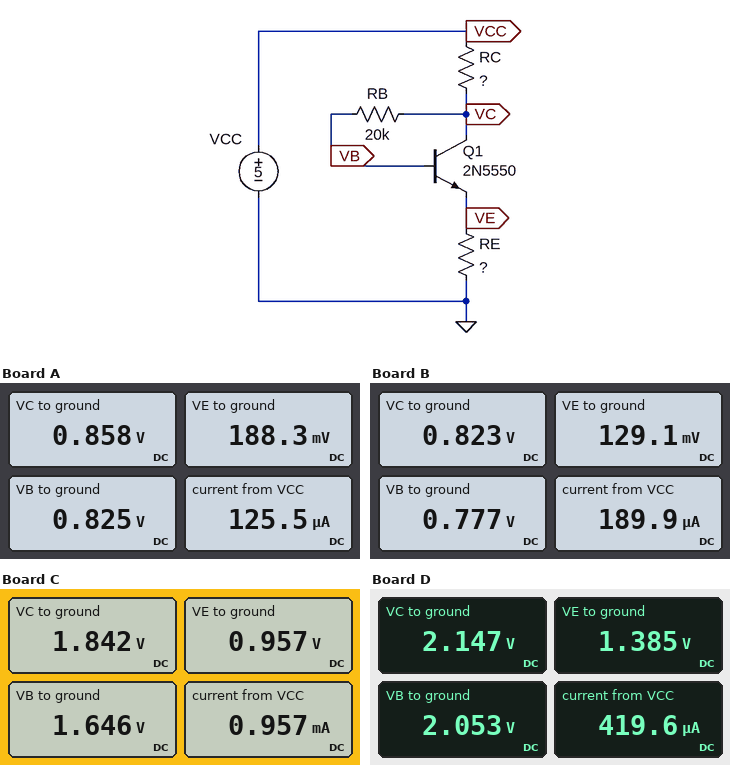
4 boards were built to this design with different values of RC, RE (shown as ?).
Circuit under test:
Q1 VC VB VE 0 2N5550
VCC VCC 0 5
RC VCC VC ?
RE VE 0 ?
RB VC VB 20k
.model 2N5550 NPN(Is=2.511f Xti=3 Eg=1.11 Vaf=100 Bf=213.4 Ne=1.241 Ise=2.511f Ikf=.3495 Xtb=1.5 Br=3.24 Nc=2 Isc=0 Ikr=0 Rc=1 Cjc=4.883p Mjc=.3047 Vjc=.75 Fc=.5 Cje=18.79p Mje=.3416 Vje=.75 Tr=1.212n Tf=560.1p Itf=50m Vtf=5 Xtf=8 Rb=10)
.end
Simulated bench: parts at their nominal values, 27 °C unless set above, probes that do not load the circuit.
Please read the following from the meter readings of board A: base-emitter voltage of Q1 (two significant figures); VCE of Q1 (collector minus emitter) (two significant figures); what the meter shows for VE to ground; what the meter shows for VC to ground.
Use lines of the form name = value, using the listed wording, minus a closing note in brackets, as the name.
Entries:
base-emitter voltage of Q1 = 640 mV
VCE of Q1 (collector minus emitter) = 670 mV
what the meter shows for VE to ground = 188.3 mV
what the meter shows for VC to ground = 0.858 V
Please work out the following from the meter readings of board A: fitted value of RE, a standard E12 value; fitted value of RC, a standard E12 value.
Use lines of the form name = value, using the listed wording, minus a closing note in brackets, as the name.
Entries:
fitted value of RE, a standard E12 value = 1.5 kΩ
fitted value of RC, a standard E12 value = 33 kΩ
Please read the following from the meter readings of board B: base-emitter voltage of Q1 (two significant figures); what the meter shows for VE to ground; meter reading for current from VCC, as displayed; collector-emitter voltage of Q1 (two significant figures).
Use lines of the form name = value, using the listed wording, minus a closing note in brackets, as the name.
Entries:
base-emitter voltage of Q1 = 650 mV
what the meter shows for VE to ground = 129.1 mV
meter reading for current from VCC, as displayed = 189.9 µA
collector-emitter voltage of Q1 = 690 mV
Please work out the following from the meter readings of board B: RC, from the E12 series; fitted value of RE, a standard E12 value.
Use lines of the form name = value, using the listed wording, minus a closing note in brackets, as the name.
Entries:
RC, from the E12 series = 22 kΩ
fitted value of RE, a standard E12 value = 680 Ω
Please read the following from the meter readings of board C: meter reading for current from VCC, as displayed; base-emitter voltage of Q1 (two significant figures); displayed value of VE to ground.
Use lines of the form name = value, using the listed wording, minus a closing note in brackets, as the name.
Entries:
meter reading for current from VCC, as displayed = 0.957 mA
base-emitter voltage of Q1 = 690 mV
displayed value of VE to ground = 0.957 V
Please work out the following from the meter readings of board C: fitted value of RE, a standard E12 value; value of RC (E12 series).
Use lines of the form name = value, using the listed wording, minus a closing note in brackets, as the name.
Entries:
fitted value of RE, a standard E12 value = 1 kΩ
value of RC = 3.3 kΩ
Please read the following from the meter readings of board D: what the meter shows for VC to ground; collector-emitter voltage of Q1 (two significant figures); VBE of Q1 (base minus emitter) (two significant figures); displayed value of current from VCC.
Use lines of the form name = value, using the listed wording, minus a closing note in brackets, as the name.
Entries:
what the meter shows for VC to ground = 2.147 V
collector-emitter voltage of Q1 = 760 mV
VBE of Q1 (base minus emitter) = 670 mV
displayed value of current from VCC = 419.6 µA
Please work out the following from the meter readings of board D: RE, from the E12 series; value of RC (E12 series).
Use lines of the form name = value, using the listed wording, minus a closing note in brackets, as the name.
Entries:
RE, from the E12 series = 3.3 kΩ
value of RC = 6.8 kΩ
